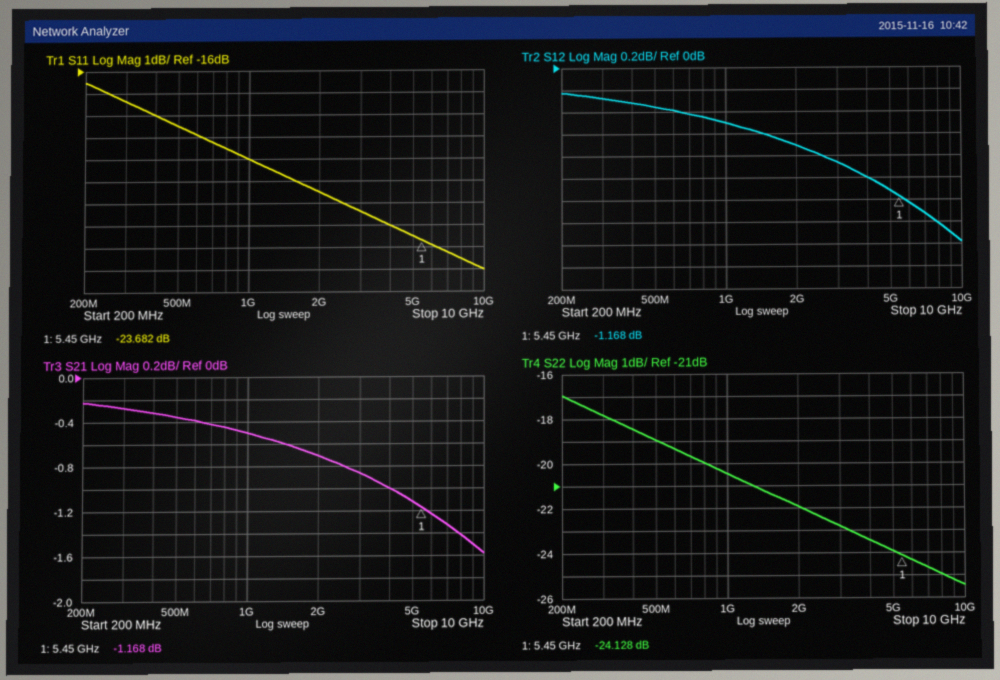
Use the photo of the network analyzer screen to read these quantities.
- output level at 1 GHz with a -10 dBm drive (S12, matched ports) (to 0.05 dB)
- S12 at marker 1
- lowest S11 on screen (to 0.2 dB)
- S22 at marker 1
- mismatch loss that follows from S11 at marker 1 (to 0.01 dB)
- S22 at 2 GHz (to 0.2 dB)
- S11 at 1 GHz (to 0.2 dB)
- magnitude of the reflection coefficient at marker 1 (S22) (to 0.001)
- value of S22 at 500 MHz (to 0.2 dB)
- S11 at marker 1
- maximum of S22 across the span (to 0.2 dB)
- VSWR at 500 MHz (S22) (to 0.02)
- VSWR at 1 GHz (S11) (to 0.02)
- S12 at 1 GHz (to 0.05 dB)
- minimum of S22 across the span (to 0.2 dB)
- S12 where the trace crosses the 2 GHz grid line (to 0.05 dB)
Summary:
-10.50 dBm
-1.168 dB
-25.0 dB
-24.128 dB
0.02 dB
-22.0 dB
-20.0 dB
0.062
-19.0 dB
-23.682 dB
-17.0 dB
1.26
1.22
-0.50 dB
-25.4 dB
-0.70 dB
